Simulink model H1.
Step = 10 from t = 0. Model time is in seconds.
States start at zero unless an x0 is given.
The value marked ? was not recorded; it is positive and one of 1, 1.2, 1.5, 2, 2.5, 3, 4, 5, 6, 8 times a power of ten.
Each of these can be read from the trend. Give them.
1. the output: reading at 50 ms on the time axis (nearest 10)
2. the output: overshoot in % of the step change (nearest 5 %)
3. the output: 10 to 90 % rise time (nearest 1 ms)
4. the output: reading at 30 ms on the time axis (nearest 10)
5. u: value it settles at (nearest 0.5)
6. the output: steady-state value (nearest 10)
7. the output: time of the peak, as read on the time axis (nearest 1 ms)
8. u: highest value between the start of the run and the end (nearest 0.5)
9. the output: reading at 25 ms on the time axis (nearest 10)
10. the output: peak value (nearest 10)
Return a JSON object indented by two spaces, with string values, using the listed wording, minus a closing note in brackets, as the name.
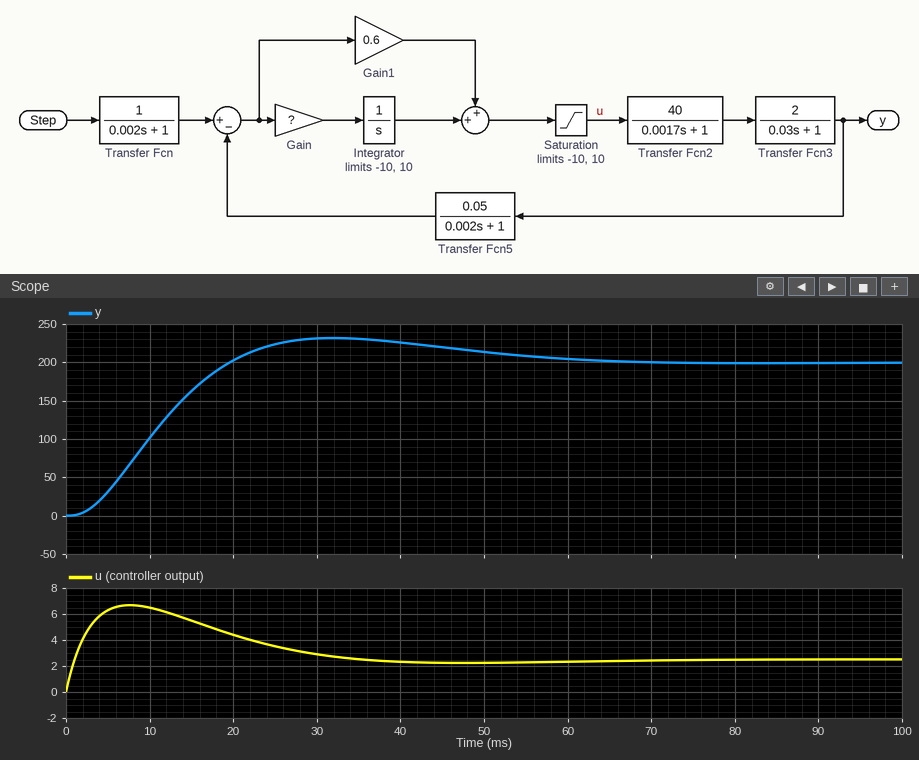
{
  "the output: reading at 50 ms on the time axis": "210",
  "the output: overshoot in % of the step change": "15 %",
  "the output: 10 to 90 % rise time": "13 ms",
  "the output: reading at 30 ms on the time axis": "230",
  "u: value it settles at": "2.5",
  "the output: steady-state value": "200",
  "the output: time of the peak, as read on the time axis": "32 ms",
  "u: highest value between the start of the run and the end": "6.5",
  "the output: reading at 25 ms on the time axis": "220",
  "the output: peak value": "230"
}
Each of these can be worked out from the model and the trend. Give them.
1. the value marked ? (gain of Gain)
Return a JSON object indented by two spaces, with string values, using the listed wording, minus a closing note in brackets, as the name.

{
  "the value marked ?": "40"
}
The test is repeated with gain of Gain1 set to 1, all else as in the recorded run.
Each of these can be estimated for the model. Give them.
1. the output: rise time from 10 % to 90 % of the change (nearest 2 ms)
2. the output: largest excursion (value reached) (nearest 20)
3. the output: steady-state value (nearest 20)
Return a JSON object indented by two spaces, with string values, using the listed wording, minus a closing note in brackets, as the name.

{
  "the output: rise time from 10 % to 90 % of the change": "10 ms",
  "the output: largest excursion (value reached)": "220",
  "the output: steady-state value": "200"
}
